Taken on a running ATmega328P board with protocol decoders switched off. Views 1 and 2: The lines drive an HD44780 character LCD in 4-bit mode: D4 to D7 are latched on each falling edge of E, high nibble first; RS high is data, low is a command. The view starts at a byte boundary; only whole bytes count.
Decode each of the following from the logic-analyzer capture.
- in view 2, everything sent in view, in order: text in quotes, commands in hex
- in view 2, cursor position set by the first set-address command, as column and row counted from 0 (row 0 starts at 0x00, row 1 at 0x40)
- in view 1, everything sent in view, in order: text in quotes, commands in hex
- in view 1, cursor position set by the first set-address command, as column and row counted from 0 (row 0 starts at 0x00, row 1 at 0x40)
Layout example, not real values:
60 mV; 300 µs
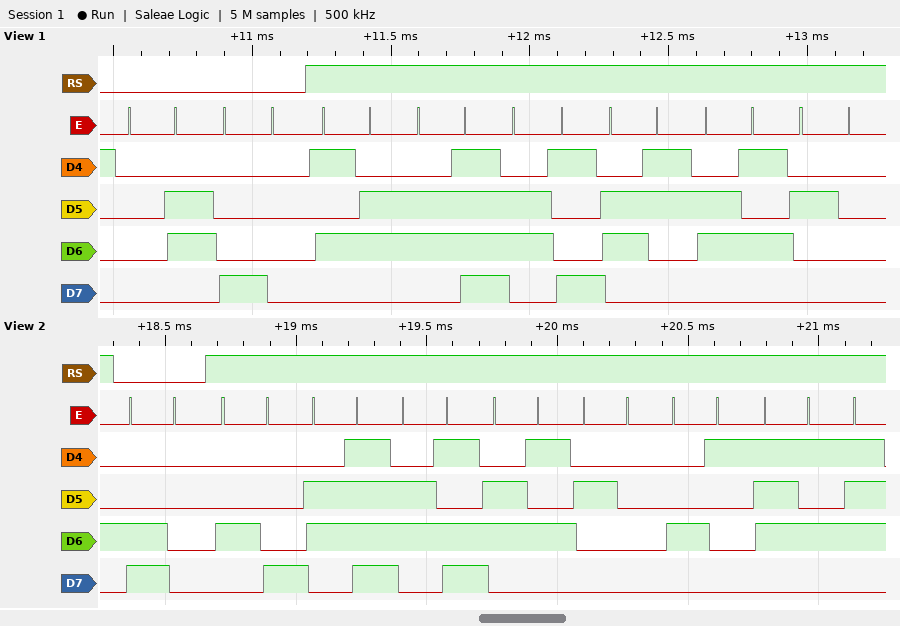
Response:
0xC0 "Home Au"; column 0, row 1; 0x06 0x80 "Voice "; column 0, row 0
